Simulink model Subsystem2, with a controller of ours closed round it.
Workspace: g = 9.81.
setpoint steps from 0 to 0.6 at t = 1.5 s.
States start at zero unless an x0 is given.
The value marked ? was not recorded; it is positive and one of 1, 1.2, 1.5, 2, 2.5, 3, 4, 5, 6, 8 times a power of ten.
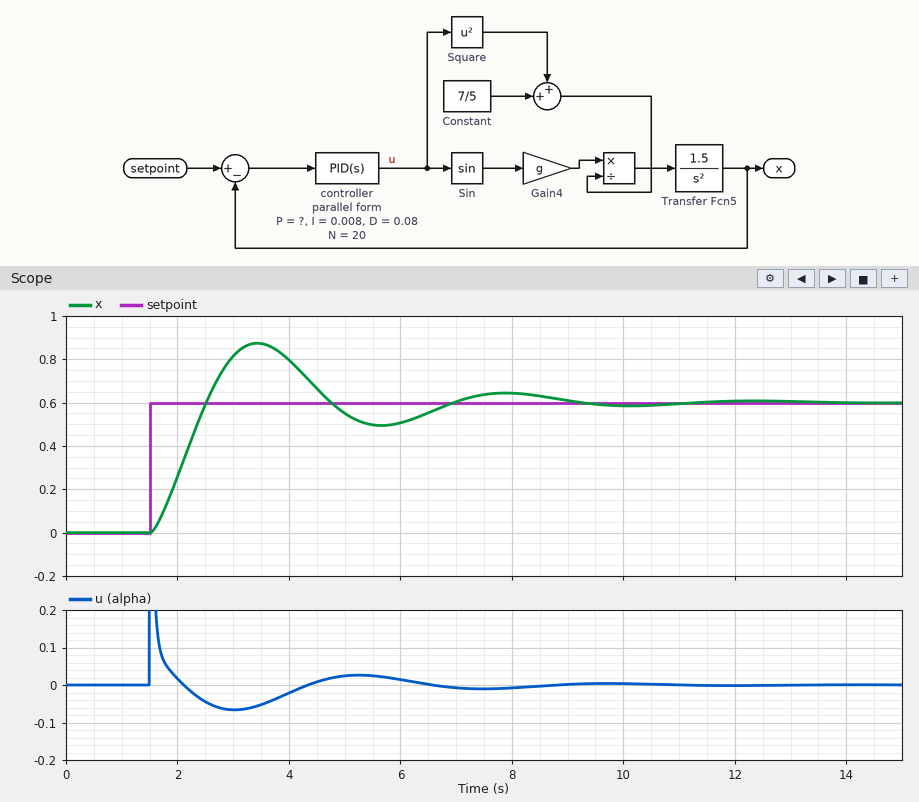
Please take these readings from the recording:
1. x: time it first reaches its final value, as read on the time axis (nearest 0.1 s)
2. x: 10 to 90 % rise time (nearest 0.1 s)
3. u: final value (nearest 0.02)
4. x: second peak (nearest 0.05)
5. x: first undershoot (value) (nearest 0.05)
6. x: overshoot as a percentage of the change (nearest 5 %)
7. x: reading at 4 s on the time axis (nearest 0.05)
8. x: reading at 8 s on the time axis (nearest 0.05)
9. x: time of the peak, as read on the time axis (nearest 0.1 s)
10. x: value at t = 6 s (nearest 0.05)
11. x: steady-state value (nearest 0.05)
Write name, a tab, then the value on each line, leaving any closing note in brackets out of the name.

x: time it first reaches its final value, as read on the time axis	2.5 s
x: 10 to 90 % rise time	0.7 s
u: final value	0.00
x: second peak	0.65
x: first undershoot (value)	0.50
x: overshoot as a percentage of the change	45 %
x: reading at 4 s on the time axis	0.80
x: reading at 8 s on the time axis	0.65
x: time of the peak, as read on the time axis	3.4 s
x: value at t = 6 s	0.50
x: steady-state value	0.60
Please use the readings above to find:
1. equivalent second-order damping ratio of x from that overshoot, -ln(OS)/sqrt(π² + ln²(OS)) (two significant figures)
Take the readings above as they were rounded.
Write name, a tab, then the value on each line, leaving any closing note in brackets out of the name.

equivalent second-order damping ratio of x from that overshoot, -ln(OS)/sqrt(π² + ln²(OS))	0.25
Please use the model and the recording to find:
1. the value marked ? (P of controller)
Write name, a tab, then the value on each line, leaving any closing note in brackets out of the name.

the value marked ?	0.2
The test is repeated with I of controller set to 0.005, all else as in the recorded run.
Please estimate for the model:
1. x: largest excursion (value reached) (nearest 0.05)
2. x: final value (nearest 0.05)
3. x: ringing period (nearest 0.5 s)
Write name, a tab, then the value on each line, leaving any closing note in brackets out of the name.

x: largest excursion (value reached)	0.85
x: final value	0.60
x: ringing period	4.5 s
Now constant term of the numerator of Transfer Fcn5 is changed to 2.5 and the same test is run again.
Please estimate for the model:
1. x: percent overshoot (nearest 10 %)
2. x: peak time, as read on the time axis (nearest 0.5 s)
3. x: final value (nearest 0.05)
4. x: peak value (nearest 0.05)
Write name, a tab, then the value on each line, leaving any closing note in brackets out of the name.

x: percent overshoot	40 %
x: peak time, as read on the time axis	3.0 s
x: final value	0.60
x: peak value	0.80
